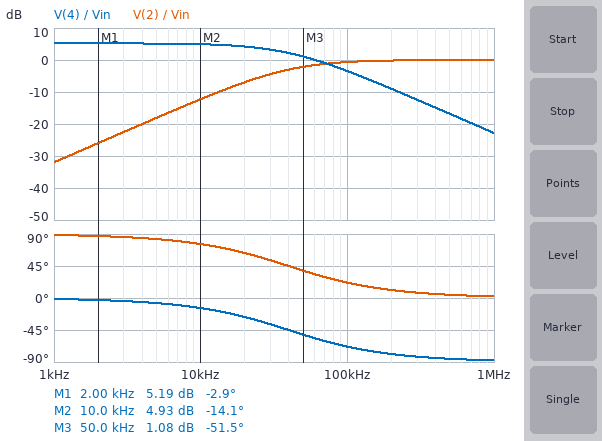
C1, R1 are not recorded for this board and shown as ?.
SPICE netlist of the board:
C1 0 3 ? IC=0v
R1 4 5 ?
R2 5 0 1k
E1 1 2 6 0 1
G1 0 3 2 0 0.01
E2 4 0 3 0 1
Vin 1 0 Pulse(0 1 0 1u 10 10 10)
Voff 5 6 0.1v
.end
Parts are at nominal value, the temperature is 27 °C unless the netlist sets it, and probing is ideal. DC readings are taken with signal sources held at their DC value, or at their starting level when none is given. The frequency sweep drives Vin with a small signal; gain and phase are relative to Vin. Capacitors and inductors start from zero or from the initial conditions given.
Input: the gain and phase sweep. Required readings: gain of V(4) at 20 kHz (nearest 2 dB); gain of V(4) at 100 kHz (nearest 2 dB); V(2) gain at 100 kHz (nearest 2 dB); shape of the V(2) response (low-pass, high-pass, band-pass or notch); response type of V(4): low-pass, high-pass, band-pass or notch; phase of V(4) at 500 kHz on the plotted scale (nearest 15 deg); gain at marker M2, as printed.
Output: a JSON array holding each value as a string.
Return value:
["4 dB", "-4 dB", "0 dB", "high-pass", "low-pass", "-90 deg", "4.93 dB"]
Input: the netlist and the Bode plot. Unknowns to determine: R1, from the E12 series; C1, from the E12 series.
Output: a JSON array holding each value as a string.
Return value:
["820 Ω", "22 nF"]
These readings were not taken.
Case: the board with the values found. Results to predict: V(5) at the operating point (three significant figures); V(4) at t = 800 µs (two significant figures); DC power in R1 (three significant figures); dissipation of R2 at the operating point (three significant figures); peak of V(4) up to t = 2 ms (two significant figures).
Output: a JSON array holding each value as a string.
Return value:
["100 mV", "2.0 V", "8.20 µW", "10.0 µW", "2.0 V"]
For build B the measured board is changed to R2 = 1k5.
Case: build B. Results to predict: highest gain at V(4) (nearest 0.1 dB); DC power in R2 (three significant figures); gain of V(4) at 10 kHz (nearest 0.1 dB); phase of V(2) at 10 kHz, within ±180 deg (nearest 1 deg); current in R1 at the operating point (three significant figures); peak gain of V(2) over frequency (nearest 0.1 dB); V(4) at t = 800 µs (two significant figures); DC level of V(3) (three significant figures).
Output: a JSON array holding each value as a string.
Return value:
["3.8 dB", "6.67 µW", "3.6 dB", "78 deg", "66.7 µA", "0 dB", "1.7 V", "155 mV"]
